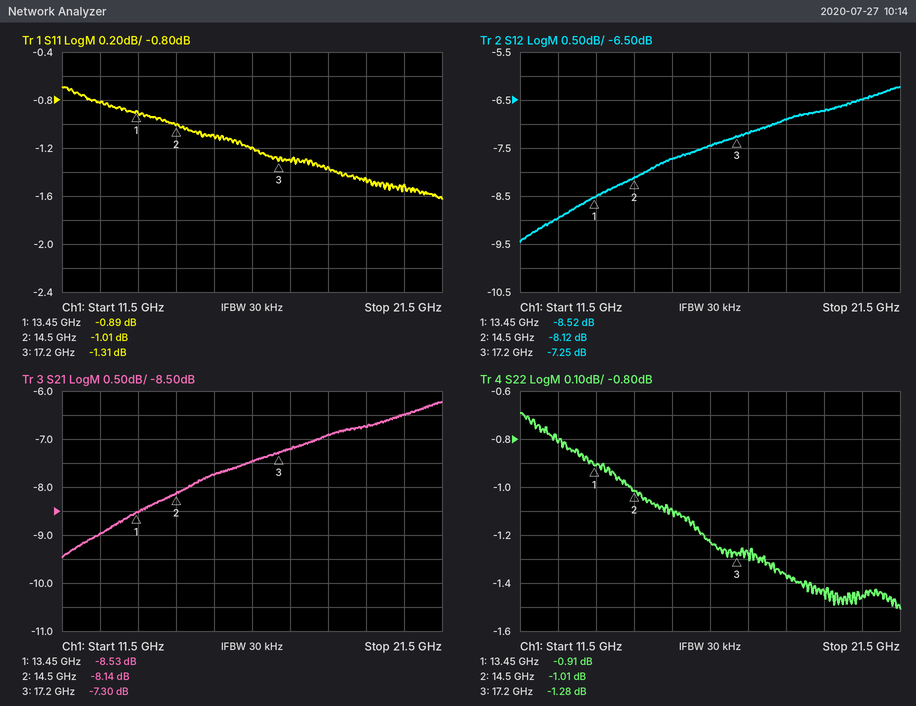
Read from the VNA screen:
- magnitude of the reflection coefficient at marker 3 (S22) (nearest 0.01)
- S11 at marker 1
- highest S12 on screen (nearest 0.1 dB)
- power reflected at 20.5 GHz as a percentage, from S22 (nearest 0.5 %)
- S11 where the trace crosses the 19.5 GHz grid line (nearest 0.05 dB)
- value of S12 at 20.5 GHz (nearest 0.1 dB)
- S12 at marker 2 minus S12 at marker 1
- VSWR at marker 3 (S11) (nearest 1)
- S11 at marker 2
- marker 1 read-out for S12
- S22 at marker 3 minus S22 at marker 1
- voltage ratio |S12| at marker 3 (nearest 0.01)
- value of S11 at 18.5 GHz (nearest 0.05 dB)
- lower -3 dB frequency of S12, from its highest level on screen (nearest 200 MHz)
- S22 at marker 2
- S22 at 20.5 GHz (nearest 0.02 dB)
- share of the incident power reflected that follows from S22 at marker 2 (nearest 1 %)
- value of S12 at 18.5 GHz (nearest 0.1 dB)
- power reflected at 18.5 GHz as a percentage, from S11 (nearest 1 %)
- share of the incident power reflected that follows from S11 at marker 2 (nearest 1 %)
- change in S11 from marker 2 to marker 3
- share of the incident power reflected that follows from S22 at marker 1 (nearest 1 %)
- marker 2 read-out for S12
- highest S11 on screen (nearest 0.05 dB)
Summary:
0.86
-0.89 dB
-6.2 dB
71.5 %
-1.45 dB
-6.5 dB
0.40 dB
13
-1.01 dB
-8.52 dB
-0.37 dB
0.43
-1.35 dB
12.0 GHz
-1.01 dB
-1.46 dB
79 %
-6.9 dB
73 %
79 %
-0.30 dB
81 %
-8.12 dB
-0.70 dB
